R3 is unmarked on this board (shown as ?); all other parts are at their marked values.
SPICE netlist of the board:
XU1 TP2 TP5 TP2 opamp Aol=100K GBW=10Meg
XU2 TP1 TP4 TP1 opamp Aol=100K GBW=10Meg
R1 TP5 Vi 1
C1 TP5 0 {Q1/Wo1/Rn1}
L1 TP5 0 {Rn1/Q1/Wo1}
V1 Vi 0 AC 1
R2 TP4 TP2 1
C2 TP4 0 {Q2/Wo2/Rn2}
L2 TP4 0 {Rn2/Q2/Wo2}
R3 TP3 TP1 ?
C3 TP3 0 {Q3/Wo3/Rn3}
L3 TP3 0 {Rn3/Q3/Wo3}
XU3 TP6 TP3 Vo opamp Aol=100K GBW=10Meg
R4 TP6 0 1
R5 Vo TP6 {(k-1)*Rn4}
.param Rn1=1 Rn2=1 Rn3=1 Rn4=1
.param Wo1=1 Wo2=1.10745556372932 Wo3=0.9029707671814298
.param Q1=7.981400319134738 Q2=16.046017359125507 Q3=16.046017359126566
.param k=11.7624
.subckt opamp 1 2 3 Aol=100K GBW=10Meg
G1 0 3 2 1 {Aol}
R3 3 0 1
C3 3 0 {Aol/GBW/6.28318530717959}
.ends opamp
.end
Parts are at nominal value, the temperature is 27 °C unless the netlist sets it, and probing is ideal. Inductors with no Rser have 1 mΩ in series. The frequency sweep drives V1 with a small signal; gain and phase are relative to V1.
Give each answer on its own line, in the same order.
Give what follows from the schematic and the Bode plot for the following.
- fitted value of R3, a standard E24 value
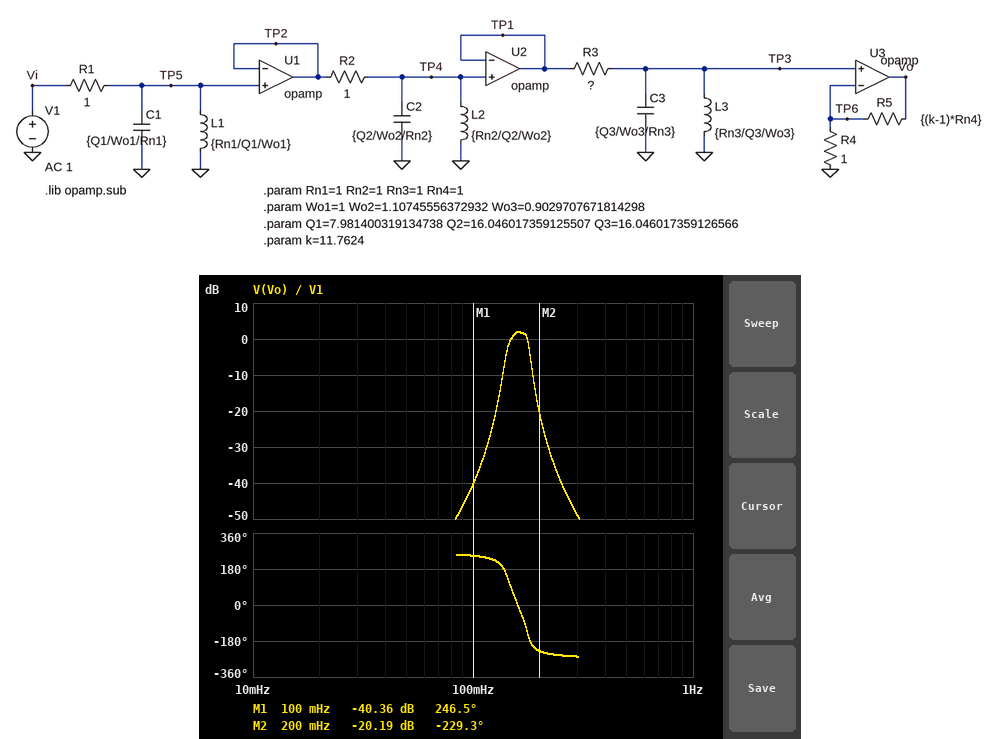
0.68 Ω
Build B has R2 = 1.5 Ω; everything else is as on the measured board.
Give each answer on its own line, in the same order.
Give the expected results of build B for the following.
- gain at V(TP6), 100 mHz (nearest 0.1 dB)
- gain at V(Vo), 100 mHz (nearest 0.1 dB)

-65.3 dB
-43.9 dB
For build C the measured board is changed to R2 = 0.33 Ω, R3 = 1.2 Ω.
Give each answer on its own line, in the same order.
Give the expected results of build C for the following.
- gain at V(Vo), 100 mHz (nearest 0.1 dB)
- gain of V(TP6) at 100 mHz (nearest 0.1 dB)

-35.7 dB
-57.1 dB
